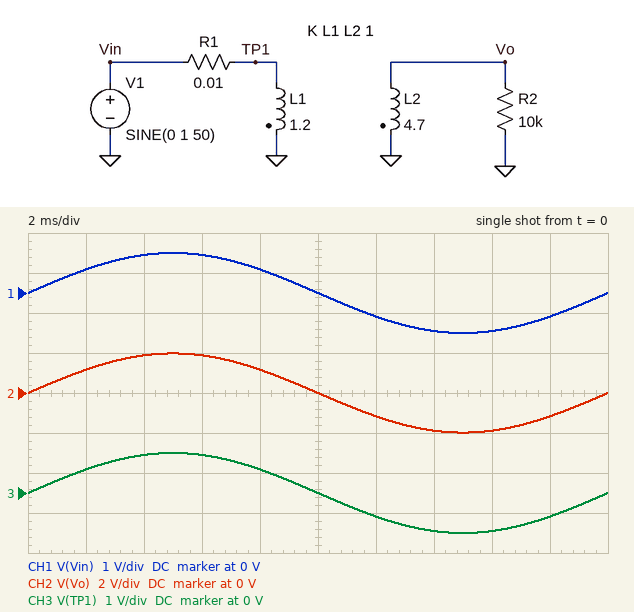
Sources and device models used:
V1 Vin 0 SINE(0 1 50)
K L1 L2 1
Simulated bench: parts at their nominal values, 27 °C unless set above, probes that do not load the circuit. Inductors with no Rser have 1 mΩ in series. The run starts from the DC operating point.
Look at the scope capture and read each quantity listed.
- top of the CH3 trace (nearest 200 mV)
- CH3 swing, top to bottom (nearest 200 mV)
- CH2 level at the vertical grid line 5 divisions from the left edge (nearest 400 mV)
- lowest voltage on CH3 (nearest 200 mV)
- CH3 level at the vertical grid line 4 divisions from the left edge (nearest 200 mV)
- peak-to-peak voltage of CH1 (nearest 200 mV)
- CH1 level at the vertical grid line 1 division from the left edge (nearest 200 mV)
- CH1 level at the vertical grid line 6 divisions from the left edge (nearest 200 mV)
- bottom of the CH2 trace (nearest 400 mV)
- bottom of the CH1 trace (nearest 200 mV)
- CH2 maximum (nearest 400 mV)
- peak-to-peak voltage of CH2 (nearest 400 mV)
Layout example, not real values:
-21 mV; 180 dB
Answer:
1.0 V; 2.0 V; 0 V; -1.0 V; 600 mV; 2.0 V; 600 mV; -600 mV; -2.0 V; -1.0 V; 2.0 V; 4.0 V
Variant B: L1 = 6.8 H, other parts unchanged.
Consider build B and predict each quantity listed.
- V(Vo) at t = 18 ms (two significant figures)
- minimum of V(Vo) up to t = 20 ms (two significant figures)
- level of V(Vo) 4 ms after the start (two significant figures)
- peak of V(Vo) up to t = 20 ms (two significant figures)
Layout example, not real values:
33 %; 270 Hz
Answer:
-490 mV; -830 mV; 790 mV; 830 mV
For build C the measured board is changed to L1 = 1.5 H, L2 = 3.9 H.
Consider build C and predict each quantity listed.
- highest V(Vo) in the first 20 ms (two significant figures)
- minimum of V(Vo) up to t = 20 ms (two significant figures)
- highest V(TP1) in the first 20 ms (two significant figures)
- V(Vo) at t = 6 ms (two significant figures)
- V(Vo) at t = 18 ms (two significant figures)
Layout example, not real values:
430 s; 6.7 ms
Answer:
1.6 V; -1.6 V; 1.0 V; 1.5 V; -950 mV
